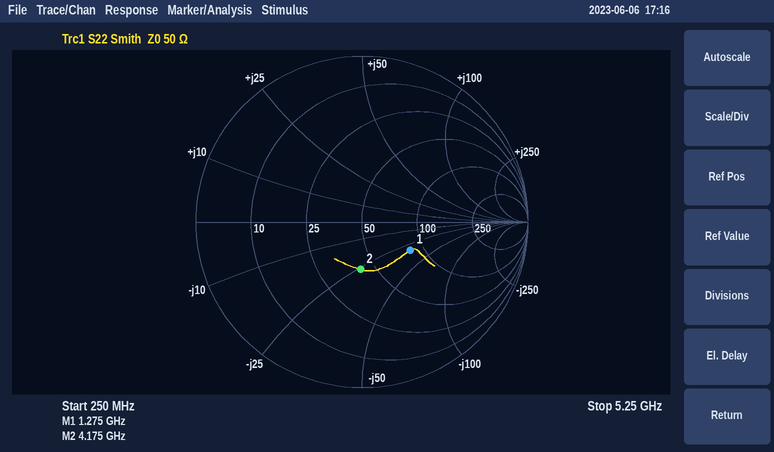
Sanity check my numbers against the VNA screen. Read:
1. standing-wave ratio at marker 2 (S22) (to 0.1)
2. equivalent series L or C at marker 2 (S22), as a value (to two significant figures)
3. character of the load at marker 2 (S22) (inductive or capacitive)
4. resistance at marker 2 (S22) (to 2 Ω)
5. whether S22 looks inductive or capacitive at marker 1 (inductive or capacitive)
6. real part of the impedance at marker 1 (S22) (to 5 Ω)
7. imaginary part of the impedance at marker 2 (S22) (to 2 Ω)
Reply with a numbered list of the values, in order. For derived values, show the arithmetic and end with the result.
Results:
1. 1.8
2. C = 1/(2π × 4.175 GHz × 26 Ω) ≈ 1.5 pF
3. capacitive
4. 42 Ω
5. capacitive
6. 85 Ω
7. -26 Ω
